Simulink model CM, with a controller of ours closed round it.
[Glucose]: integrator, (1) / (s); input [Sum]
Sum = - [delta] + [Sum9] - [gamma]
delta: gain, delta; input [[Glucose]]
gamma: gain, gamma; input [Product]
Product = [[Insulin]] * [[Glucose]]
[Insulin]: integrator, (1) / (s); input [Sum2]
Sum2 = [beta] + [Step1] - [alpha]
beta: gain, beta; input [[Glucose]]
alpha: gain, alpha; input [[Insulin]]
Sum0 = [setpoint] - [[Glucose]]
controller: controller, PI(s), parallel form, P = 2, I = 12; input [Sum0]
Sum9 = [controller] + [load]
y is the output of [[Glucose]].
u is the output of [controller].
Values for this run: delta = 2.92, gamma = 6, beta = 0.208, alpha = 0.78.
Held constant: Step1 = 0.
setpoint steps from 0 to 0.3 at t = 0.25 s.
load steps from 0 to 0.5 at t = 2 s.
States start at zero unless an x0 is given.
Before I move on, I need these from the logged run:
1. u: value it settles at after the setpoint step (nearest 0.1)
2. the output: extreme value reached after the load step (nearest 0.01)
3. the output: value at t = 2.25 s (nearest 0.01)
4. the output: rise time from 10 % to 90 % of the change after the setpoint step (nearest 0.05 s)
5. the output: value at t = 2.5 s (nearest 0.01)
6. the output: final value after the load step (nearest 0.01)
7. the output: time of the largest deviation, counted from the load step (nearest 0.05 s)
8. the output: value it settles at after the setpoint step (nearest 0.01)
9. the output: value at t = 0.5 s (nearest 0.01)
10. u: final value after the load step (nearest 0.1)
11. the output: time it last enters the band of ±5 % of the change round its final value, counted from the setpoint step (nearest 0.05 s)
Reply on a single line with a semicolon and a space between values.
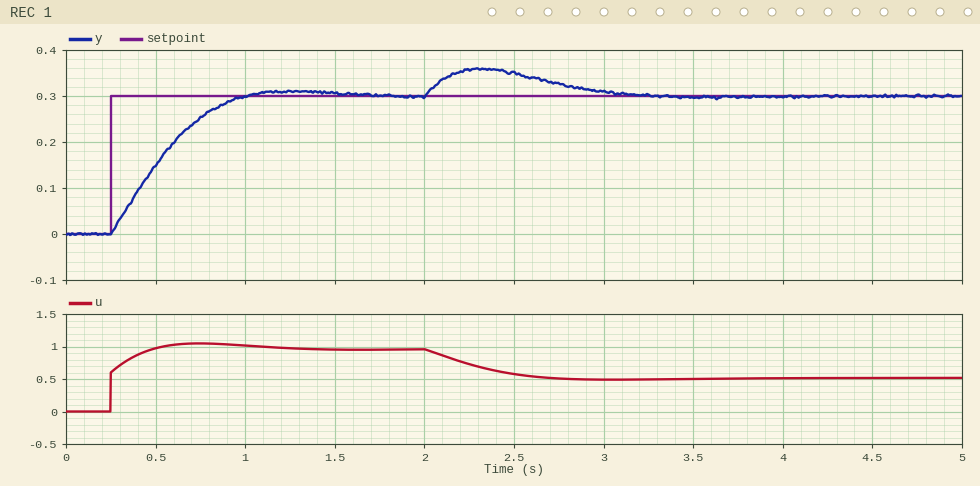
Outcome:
1.0; 0.36; 0.36; 0.50 s; 0.35; 0.30; 0.30 s; 0.30; 0.15; 0.5; 0.65 s
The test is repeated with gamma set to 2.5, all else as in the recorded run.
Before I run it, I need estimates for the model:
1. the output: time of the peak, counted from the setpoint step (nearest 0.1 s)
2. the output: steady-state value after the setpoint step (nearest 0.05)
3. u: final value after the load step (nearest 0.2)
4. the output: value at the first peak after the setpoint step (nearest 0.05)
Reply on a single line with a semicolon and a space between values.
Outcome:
1.0 s; 0.30; 0.4; 0.30
